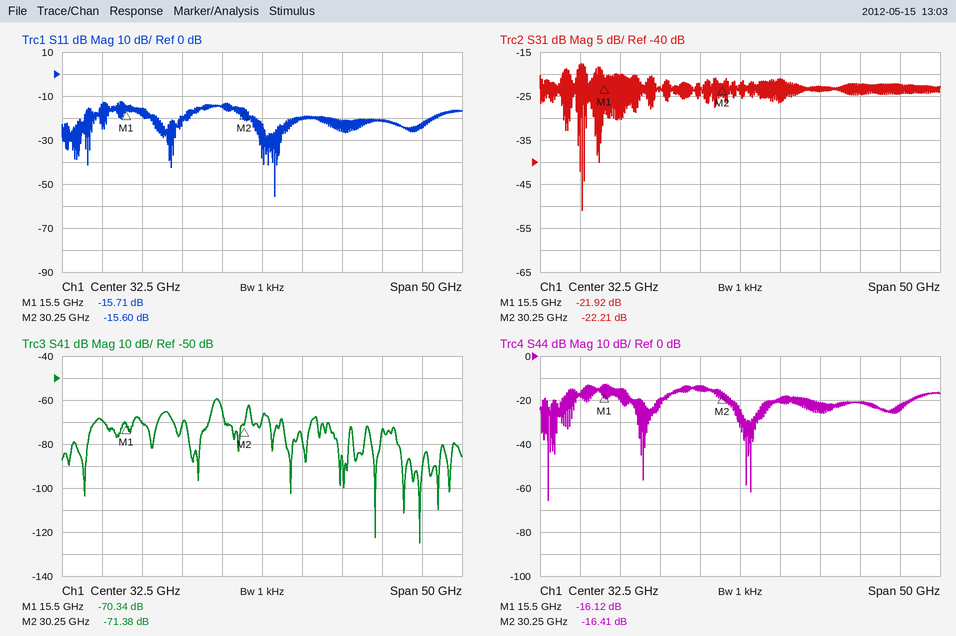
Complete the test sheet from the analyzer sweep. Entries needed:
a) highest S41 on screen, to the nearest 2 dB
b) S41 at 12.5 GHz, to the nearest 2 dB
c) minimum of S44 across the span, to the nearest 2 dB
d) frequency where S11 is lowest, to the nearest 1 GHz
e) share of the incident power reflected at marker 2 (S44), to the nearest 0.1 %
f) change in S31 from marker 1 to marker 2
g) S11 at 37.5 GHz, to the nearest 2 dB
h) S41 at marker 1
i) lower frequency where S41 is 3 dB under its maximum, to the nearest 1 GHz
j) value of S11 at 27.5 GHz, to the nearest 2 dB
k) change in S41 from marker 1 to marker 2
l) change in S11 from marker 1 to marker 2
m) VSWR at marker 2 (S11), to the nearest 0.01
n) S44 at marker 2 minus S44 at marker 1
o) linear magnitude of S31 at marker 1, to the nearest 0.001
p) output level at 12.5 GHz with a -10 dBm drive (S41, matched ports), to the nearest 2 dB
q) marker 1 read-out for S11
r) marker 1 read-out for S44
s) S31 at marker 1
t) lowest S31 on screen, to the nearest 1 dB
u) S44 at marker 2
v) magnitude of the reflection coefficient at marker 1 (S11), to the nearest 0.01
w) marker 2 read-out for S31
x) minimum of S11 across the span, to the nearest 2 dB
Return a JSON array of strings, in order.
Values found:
["-60 dB", "-70 dB", "-66 dB", "34 GHz", "2.3 %", "-0.29 dB", "-20 dB", "-70.34 dB", "26 GHz", "-14 dB", "-1.04 dB", "0.11 dB", "1.40", "-0.29 dB", "0.080", "-80 dBm", "-15.71 dB", "-16.12 dB", "-21.92 dB", "-51 dB", "-16.41 dB", "0.16", "-22.21 dB", "-56 dB"]
